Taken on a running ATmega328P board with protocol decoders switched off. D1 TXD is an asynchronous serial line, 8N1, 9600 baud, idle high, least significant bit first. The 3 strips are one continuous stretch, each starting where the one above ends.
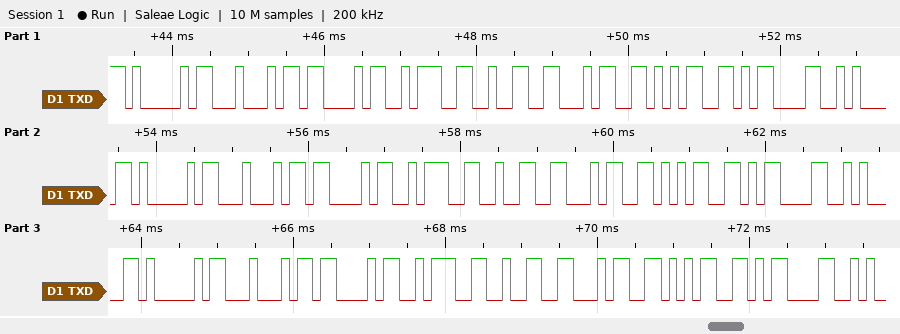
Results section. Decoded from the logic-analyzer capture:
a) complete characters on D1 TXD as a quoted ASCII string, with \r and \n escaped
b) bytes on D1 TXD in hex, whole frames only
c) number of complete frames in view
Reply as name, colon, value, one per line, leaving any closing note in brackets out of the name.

complete characters on D1 TXD as a quoted ASCII string, with \r and \n escaped: "ADC:245\r\nADC:245\r\nADC:245\r"
bytes on D1 TXD in hex, whole frames only: 41 44 43 3A 32 34 35 0D 0A 41 44 43 3A 32 34 35 0D 0A 41 44 43 3A 32 34 35 0D
number of complete frames in view: 26
